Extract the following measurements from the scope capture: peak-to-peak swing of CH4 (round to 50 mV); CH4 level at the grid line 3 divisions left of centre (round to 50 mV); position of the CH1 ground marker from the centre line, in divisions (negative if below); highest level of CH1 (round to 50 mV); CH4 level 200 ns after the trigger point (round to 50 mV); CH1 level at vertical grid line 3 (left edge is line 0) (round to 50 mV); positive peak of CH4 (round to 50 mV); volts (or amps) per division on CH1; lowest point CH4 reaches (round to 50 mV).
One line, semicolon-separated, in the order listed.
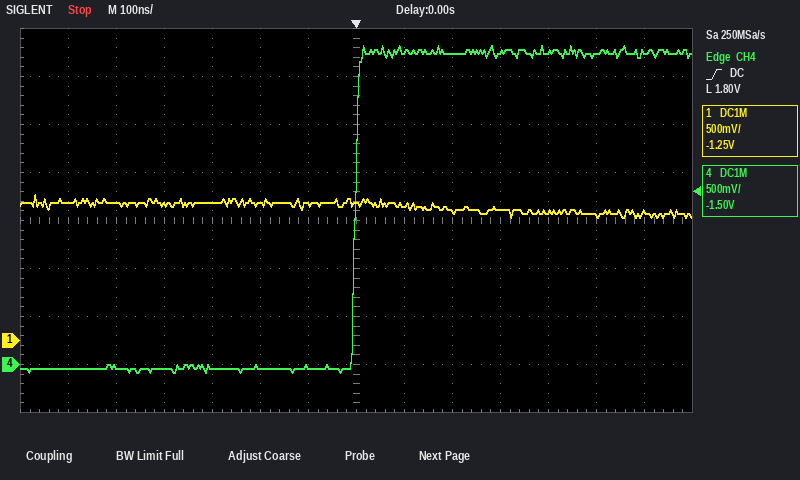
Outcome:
3.40 V; -50 mV; -2.5 div; 1.50 V; 3.25 V; 1.40 V; 3.30 V; 500 mV; -100 mV
